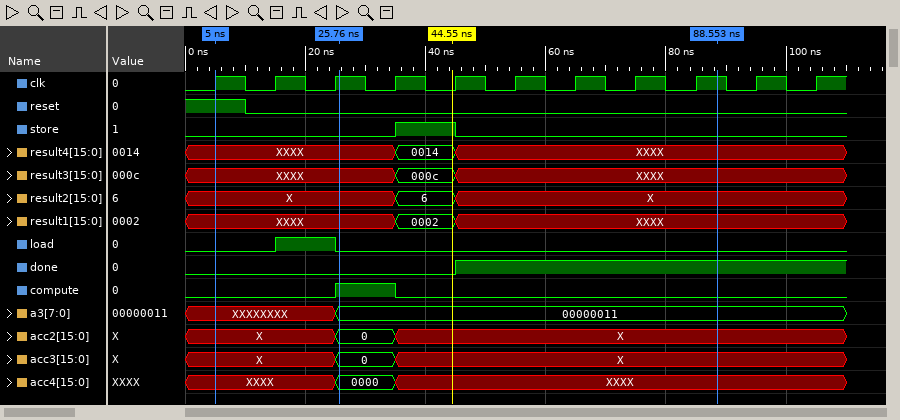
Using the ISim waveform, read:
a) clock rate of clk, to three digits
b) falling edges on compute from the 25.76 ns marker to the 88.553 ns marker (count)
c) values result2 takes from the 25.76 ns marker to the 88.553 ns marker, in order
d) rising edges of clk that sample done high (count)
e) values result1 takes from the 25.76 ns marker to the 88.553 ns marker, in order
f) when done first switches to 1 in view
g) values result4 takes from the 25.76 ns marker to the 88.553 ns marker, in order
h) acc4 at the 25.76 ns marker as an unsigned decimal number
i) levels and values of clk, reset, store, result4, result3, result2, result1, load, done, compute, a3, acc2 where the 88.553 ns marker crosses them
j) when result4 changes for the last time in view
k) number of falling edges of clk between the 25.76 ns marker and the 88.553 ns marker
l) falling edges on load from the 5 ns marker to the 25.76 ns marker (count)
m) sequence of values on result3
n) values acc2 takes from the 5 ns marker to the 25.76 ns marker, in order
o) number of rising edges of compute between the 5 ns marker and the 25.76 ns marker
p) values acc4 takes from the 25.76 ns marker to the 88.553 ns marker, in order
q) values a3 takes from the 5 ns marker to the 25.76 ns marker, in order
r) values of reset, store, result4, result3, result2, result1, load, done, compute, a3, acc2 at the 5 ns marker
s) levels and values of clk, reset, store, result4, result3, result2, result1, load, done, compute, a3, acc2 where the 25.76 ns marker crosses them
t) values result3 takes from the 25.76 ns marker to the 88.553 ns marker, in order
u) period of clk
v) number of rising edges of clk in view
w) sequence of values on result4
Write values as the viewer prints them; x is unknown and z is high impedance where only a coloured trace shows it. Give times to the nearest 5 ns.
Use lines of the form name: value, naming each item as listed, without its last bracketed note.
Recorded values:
clock rate of clk, to three digits: 100 MHz
falling edges on compute from the 25.76 ns marker to the 88.553 ns marker: 1
values result2 takes from the 25.76 ns marker to the 88.553 ns marker, in order: X, 6, X
rising edges of clk that sample done high: 6
values result1 takes from the 25.76 ns marker to the 88.553 ns marker, in order: XXXX, 0002, XXXX
when done first switches to 1 in view: 45 ns
values result4 takes from the 25.76 ns marker to the 88.553 ns marker, in order: XXXX, 0014, XXXX
acc4 at the 25.76 ns marker as an unsigned decimal number: 0
levels and values of clk, reset, store, result4, result3, result2, result1, load, done, compute, a3, acc2 where the 88.553 ns marker crosses them: clk=1, reset=0, store=0, result4=XXXX, result3=XXXX, result2=X, result1=XXXX, load=0, done=1, compute=0, a3=00000011, acc2=X
when result4 changes for the last time in view: 45 ns
number of falling edges of clk between the 25.76 ns marker and the 88.553 ns marker: 6
falling edges on load from the 5 ns marker to the 25.76 ns marker: 1
sequence of values on result3: XXXX, 000c, XXXX
values acc2 takes from the 5 ns marker to the 25.76 ns marker, in order: X, 0
number of rising edges of compute between the 5 ns marker and the 25.76 ns marker: 1
values acc4 takes from the 25.76 ns marker to the 88.553 ns marker, in order: 0000, XXXX
values a3 takes from the 5 ns marker to the 25.76 ns marker, in order: XXXXXXXX, 00000011
values of reset, store, result4, result3, result2, result1, load, done, compute, a3, acc2 at the 5 ns marker: reset=1, store=0, result4=XXXX, result3=XXXX, result2=X, result1=XXXX, load=0, done=0, compute=0, a3=XXXXXXXX, acc2=X
levels and values of clk, reset, store, result4, result3, result2, result1, load, done, compute, a3, acc2 where the 25.76 ns marker crosses them: clk=1, reset=0, store=0, result4=XXXX, result3=XXXX, result2=X, result1=XXXX, load=0, done=0, compute=1, a3=00000011, acc2=0
values result3 takes from the 25.76 ns marker to the 88.553 ns marker, in order: XXXX, 000c, XXXX
period of clk: 10 ns
number of rising edges of clk in view: 11
sequence of values on result4: XXXX, 0014, XXXX
